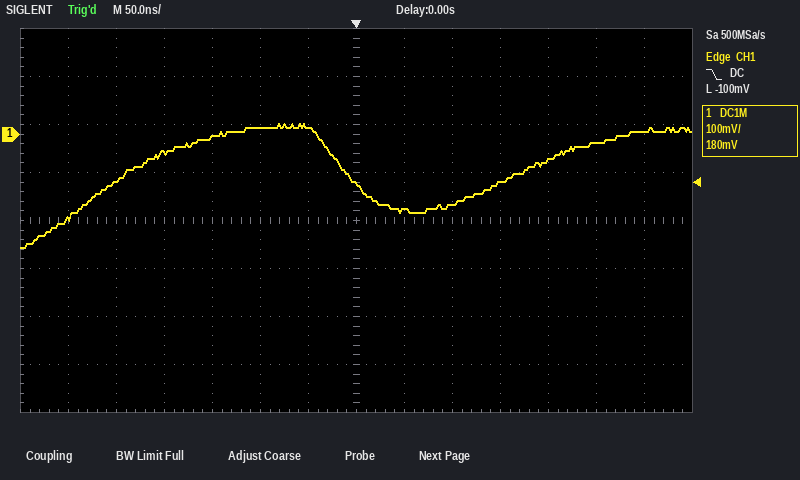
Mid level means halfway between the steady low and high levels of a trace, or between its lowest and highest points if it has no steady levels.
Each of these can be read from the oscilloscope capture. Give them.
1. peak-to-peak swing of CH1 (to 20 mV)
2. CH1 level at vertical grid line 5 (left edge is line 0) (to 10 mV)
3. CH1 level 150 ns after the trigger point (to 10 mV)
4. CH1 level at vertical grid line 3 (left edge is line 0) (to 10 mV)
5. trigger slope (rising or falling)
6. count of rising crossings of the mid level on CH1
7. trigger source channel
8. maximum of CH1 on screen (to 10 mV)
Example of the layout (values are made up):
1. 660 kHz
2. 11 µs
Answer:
1. 260 mV
2. 10 mV
3. -100 mV
4. -40 mV
5. falling
6. 2
7. CH1
8. 20 mV
